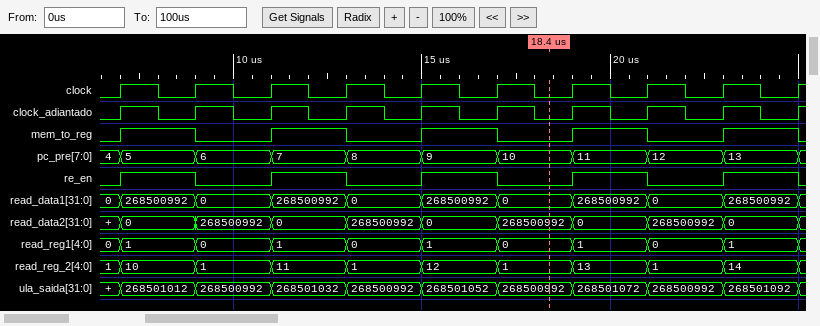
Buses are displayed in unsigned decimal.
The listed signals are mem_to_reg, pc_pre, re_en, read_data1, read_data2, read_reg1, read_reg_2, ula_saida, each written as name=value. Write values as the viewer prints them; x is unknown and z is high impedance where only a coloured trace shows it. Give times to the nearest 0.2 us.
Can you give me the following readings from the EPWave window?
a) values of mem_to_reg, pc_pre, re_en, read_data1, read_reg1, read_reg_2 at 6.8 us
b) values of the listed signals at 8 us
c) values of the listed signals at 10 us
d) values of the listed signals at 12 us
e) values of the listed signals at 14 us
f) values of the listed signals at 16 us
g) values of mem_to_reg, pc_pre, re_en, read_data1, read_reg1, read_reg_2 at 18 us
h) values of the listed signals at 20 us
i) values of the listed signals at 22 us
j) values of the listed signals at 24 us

mem_to_reg=0, pc_pre=4, re_en=0, read_data1=0, read_reg1=0, read_reg_2=1
mem_to_reg=1, pc_pre=5, re_en=1, read_data1=268500992, read_data2=0, read_reg1=1, read_reg_2=10, ula_saida=268501012
mem_to_reg=0, pc_pre=6, re_en=0, read_data1=0, read_data2=268500992, read_reg1=0, read_reg_2=1, ula_saida=268500992
mem_to_reg=1, pc_pre=7, re_en=1, read_data1=268500992, read_data2=0, read_reg1=1, read_reg_2=11, ula_saida=268501032
mem_to_reg=0, pc_pre=8, re_en=0, read_data1=0, read_data2=268500992, read_reg1=0, read_reg_2=1, ula_saida=268500992
mem_to_reg=1, pc_pre=9, re_en=1, read_data1=268500992, read_data2=0, read_reg1=1, read_reg_2=12, ula_saida=268501052
mem_to_reg=0, pc_pre=10, re_en=0, read_data1=0, read_reg1=0, read_reg_2=1
mem_to_reg=1, pc_pre=11, re_en=1, read_data1=268500992, read_data2=0, read_reg1=1, read_reg_2=13, ula_saida=268501072
mem_to_reg=0, pc_pre=12, re_en=0, read_data1=0, read_data2=268500992, read_reg1=0, read_reg_2=1, ula_saida=268500992
mem_to_reg=1, pc_pre=13, re_en=1, read_data1=268500992, read_data2=0, read_reg1=1, read_reg_2=14, ula_saida=268501092
